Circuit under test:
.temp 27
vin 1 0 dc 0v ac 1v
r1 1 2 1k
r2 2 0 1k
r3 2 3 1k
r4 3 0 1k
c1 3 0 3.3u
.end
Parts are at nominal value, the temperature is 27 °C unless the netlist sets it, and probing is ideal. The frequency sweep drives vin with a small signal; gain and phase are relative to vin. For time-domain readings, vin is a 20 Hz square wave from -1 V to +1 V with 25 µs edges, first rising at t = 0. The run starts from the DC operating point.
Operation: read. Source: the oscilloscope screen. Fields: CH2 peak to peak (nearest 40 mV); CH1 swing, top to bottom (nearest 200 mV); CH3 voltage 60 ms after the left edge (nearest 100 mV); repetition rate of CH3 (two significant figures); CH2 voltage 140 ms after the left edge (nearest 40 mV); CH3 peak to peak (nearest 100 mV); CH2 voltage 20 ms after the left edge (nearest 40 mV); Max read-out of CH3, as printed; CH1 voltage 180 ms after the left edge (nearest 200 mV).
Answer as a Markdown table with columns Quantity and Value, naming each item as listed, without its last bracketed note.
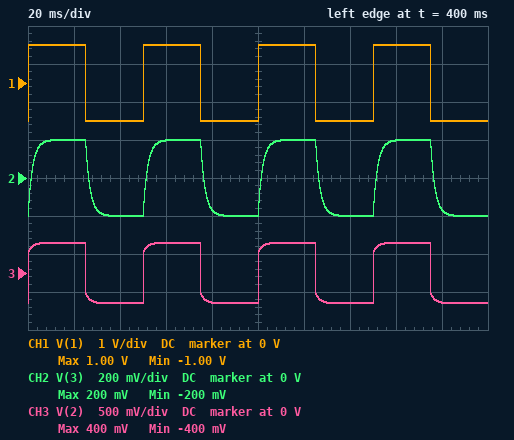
| Quantity | Value |
|---|---|
| CH2 peak to peak | 400 mV |
| CH1 swing, top to bottom | 2.0 V |
| CH3 voltage 60 ms after the left edge | 400 mV |
| repetition rate of CH3 | 20 Hz |
| CH2 voltage 140 ms after the left edge | -200 mV |
| CH3 peak to peak | 800 mV |
| CH2 voltage 20 ms after the left edge | 200 mV |
| Max read-out of CH3, as printed | 400 mV |
| CH1 voltage 180 ms after the left edge | -1.0 V |
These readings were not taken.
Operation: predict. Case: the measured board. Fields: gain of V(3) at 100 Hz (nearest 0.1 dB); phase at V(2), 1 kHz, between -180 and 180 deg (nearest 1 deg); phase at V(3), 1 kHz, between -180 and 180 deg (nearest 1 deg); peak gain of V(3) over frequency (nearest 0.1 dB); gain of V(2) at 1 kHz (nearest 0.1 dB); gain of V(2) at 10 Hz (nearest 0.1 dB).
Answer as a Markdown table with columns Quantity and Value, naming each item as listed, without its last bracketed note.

| Quantity | Value |
|---|---|
| gain of V(3) at 100 Hz | -18.0 dB |
| phase at V(2), 1 kHz, between -180 and 180 deg | -1 deg |
| phase at V(3), 1 kHz, between -180 and 180 deg | -85 deg |
| peak gain of V(3) over frequency | -14.0 dB |
| gain of V(2) at 1 kHz | -9.5 dB |
| gain of V(2) at 10 Hz | -8.0 dB |
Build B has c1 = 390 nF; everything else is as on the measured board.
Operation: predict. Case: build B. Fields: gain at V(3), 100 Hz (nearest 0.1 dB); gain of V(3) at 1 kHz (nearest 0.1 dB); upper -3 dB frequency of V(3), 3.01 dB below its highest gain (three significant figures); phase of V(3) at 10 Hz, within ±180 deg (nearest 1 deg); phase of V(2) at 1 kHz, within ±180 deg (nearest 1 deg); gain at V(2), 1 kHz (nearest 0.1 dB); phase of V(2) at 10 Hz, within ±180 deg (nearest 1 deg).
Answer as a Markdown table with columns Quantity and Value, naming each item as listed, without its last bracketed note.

| Quantity | Value |
|---|---|
| gain at V(3), 100 Hz | -14.1 dB |
| gain of V(3) at 1 kHz | -19.0 dB |
| upper -3 dB frequency of V(3), 3.01 dB below its highest gain | 680 Hz |
| phase of V(3) at 10 Hz, within ±180 deg | -1 deg |
| phase of V(2) at 1 kHz, within ±180 deg | -5 deg |
| gain at V(2), 1 kHz | -9.0 dB |
| phase of V(2) at 10 Hz, within ±180 deg | 0 deg |
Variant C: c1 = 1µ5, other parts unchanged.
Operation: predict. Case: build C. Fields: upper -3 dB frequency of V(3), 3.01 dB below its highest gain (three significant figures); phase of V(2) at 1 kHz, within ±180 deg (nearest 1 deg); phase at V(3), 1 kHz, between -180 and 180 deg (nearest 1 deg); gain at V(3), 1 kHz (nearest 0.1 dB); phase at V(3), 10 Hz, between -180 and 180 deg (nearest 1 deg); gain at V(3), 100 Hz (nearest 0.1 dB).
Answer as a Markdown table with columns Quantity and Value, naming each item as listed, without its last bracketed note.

| Quantity | Value |
|---|---|
| upper -3 dB frequency of V(3), 3.01 dB below its highest gain | 177 Hz |
| phase of V(2) at 1 kHz, within ±180 deg | -2 deg |
| phase at V(3), 1 kHz, between -180 and 180 deg | -80 deg |
| gain at V(3), 1 kHz | -29.2 dB |
| phase at V(3), 10 Hz, between -180 and 180 deg | -3 deg |
| gain at V(3), 100 Hz | -15.2 dB |
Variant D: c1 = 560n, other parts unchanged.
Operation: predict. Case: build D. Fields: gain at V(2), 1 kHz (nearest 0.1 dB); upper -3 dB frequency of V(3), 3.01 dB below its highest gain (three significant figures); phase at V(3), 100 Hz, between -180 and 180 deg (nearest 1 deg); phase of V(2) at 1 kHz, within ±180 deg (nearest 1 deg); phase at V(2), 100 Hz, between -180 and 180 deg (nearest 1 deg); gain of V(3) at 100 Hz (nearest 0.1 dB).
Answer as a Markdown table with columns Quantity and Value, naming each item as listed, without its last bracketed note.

| Quantity | Value |
|---|---|
| gain at V(2), 1 kHz | -9.2 dB |
| upper -3 dB frequency of V(3), 3.01 dB below its highest gain | 474 Hz |
| phase at V(3), 100 Hz, between -180 and 180 deg | -12 deg |
| phase of V(2) at 1 kHz, within ±180 deg | -4 deg |
| phase at V(2), 100 Hz, between -180 and 180 deg | -2 deg |
| gain of V(3) at 100 Hz | -14.2 dB |
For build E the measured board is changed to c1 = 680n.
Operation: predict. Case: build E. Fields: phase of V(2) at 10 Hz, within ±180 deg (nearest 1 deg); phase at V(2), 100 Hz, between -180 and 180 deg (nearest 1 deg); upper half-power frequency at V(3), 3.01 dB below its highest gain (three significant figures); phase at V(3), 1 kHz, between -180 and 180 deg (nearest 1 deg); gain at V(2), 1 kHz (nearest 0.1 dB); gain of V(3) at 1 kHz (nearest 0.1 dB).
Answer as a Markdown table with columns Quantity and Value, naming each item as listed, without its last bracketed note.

| Quantity | Value |
|---|---|
| phase of V(2) at 10 Hz, within ±180 deg | 0 deg |
| phase at V(2), 100 Hz, between -180 and 180 deg | -2 deg |
| upper half-power frequency at V(3), 3.01 dB below its highest gain | 390 Hz |
| phase at V(3), 1 kHz, between -180 and 180 deg | -69 deg |
| gain at V(2), 1 kHz | -9.3 dB |
| gain of V(3) at 1 kHz | -22.8 dB |
